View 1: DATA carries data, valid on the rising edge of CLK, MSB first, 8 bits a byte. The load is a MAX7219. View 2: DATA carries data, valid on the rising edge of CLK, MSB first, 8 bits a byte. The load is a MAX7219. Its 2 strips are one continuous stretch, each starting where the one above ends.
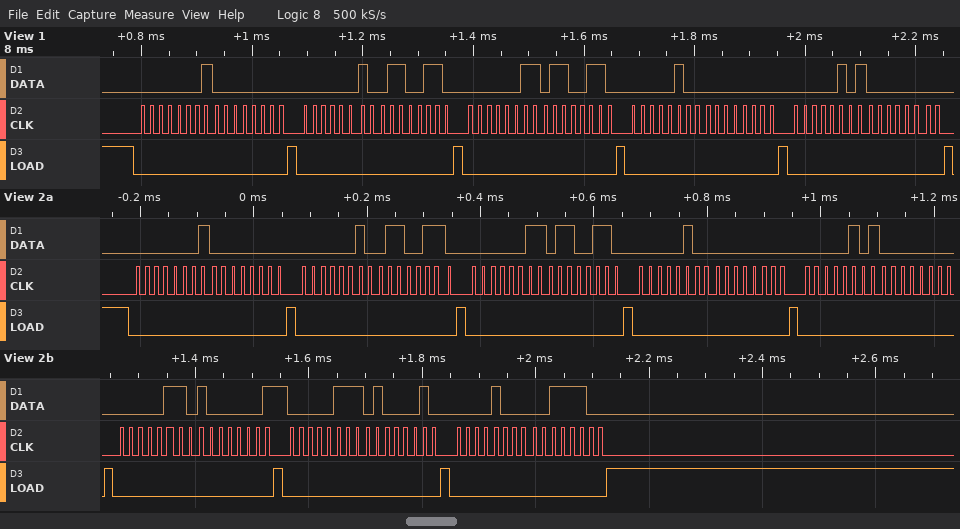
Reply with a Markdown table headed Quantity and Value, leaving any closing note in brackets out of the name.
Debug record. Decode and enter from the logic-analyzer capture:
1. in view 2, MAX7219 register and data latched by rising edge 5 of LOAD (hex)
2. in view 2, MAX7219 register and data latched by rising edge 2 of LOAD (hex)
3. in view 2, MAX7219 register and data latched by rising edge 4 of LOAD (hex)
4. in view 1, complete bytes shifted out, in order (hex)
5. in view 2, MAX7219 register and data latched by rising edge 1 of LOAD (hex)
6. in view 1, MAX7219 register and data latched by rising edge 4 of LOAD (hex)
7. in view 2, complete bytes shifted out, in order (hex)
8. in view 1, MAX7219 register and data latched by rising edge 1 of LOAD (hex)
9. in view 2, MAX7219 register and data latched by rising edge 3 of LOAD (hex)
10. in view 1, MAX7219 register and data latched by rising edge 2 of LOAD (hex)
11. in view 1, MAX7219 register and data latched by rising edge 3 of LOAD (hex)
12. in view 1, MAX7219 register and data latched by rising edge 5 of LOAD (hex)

| Quantity | Value |
|---|---|
| in view 2, MAX7219 register and data latched by rising edge 5 of LOAD | register 0x5, data 0x00 |
| in view 2, MAX7219 register and data latched by rising edge 2 of LOAD | register 0x2, data 0x66 |
| in view 2, MAX7219 register and data latched by rising edge 4 of LOAD | register 0x4, data 0x00 |
| in view 1, complete bytes shifted out, in order | 01 00 02 66 03 66 04 00 05 00 |
| in view 2, MAX7219 register and data latched by rising edge 1 of LOAD | register 0x1, data 0x00 |
| in view 1, MAX7219 register and data latched by rising edge 4 of LOAD | register 0x4, data 0x00 |
| in view 2, complete bytes shifted out, in order | 01 00 02 66 03 66 04 00 05 00 06 81 07 42 08 3C |
| in view 1, MAX7219 register and data latched by rising edge 1 of LOAD | register 0x1, data 0x00 |
| in view 2, MAX7219 register and data latched by rising edge 3 of LOAD | register 0x3, data 0x66 |
| in view 1, MAX7219 register and data latched by rising edge 2 of LOAD | register 0x2, data 0x66 |
| in view 1, MAX7219 register and data latched by rising edge 3 of LOAD | register 0x3, data 0x66 |
| in view 1, MAX7219 register and data latched by rising edge 5 of LOAD | register 0x5, data 0x00 |
